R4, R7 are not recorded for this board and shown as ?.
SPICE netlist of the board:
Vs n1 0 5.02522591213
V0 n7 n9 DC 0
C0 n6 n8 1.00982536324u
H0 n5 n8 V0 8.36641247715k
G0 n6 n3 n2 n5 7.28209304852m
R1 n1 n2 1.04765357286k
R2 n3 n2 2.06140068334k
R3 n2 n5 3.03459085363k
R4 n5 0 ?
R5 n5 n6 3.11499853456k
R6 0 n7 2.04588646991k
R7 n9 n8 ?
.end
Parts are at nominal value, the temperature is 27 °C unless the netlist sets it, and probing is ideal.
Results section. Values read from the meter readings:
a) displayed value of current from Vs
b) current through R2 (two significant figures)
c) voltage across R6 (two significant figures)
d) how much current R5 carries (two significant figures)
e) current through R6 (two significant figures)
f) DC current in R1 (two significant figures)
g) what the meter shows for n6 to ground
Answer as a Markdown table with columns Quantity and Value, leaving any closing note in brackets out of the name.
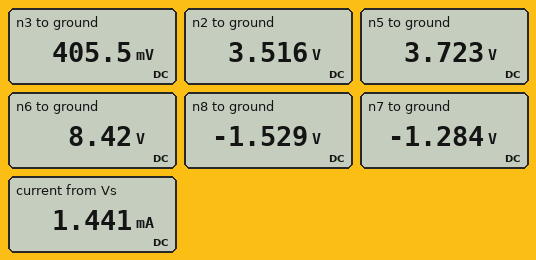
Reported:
| Quantity | Value |
|---|---|
| displayed value of current from Vs | 1.441 mA |
| current through R2 | 1.5 mA |
| voltage across R6 | 1.3 V |
| how much current R5 carries | 1.5 mA |
| current through R6 | 630 µA |
| DC current in R1 | 1.4 mA |
| what the meter shows for n6 to ground | 8.42 V |
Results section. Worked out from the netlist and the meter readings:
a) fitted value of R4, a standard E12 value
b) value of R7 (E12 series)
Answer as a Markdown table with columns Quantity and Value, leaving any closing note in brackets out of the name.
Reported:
| Quantity | Value |
|---|---|
| fitted value of R4, a standard E12 value | 1.8 kΩ |
| value of R7 | 390 Ω |
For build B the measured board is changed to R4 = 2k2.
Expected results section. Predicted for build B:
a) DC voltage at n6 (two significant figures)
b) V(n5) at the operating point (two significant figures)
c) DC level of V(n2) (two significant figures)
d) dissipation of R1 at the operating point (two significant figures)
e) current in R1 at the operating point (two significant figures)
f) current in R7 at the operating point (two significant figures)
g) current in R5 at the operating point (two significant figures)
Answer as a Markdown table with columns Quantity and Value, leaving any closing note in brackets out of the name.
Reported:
| Quantity | Value |
|---|---|
| DC voltage at n6 | 7.7 V |
| V(n5) at the operating point | 4.0 V |
| DC level of V(n2) | 3.8 V |
| dissipation of R1 at the operating point | 1.4 mW |
| current in R1 at the operating point | 1.1 mA |
| current in R7 at the operating point | 670 µA |
| current in R5 at the operating point | 1.2 mA |
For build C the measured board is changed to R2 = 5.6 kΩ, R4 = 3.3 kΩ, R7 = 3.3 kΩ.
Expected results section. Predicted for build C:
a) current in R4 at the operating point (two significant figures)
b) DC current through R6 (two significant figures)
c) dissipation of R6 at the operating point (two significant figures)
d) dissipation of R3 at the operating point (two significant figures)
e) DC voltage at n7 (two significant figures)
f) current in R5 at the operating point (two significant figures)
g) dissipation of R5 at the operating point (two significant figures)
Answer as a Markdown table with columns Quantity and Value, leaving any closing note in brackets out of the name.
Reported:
| Quantity | Value |
|---|---|
| current in R4 at the operating point | 1.6 mA |
| DC current through R6 | 1.7 mA |
| dissipation of R6 at the operating point | 6.0 mW |
| dissipation of R3 at the operating point | 140 nW |
| DC voltage at n7 | -3.5 V |
| current in R5 at the operating point | 150 µA |
| dissipation of R5 at the operating point | 71 µW |
